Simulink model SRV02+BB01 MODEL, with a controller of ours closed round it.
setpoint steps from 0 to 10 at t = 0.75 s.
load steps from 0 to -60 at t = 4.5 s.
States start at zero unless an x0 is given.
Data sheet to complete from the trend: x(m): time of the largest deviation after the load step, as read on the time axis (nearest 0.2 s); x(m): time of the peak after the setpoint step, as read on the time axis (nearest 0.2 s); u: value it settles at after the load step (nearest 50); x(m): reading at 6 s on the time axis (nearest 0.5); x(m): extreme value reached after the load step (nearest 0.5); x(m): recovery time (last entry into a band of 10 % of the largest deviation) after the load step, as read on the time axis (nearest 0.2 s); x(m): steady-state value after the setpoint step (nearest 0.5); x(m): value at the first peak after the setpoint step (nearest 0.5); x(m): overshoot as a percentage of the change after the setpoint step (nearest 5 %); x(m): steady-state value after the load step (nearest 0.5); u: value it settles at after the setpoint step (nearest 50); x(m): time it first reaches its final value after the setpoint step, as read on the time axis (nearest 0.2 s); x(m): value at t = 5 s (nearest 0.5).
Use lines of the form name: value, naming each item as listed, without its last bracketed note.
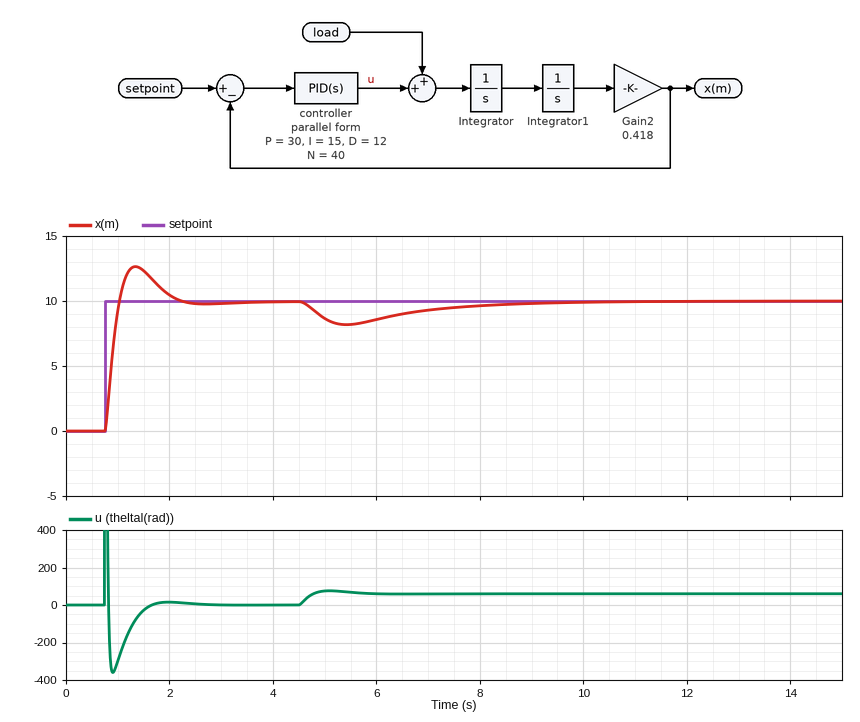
x(m): time of the largest deviation after the load step, as read on the time axis: 5.4 s
x(m): time of the peak after the setpoint step, as read on the time axis: 1.4 s
u: value it settles at after the load step: 50
x(m): reading at 6 s on the time axis: 8.5
x(m): extreme value reached after the load step: 8.0
x(m): recovery time (last entry into a band of 10 % of the largest deviation) after the load step, as read on the time axis: 9.2 s
x(m): steady-state value after the setpoint step: 10.0
x(m): value at the first peak after the setpoint step: 12.5
x(m): overshoot as a percentage of the change after the setpoint step: 25 %
x(m): steady-state value after the load step: 10.0
u: value it settles at after the setpoint step: 0
x(m): time it first reaches its final value after the setpoint step, as read on the time axis: 1.0 s
x(m): value at t = 5 s: 8.5
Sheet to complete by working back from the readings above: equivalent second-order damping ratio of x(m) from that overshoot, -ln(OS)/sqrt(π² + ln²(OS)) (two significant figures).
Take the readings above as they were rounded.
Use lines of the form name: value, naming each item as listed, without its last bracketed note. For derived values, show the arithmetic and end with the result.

equivalent second-order damping ratio of x(m) from that overshoot, -ln(OS)/sqrt(π² + ln²(OS)): ln(0.25) = -1.386; 1.386 / sqrt(9.870 + 1.922) = 0.40
